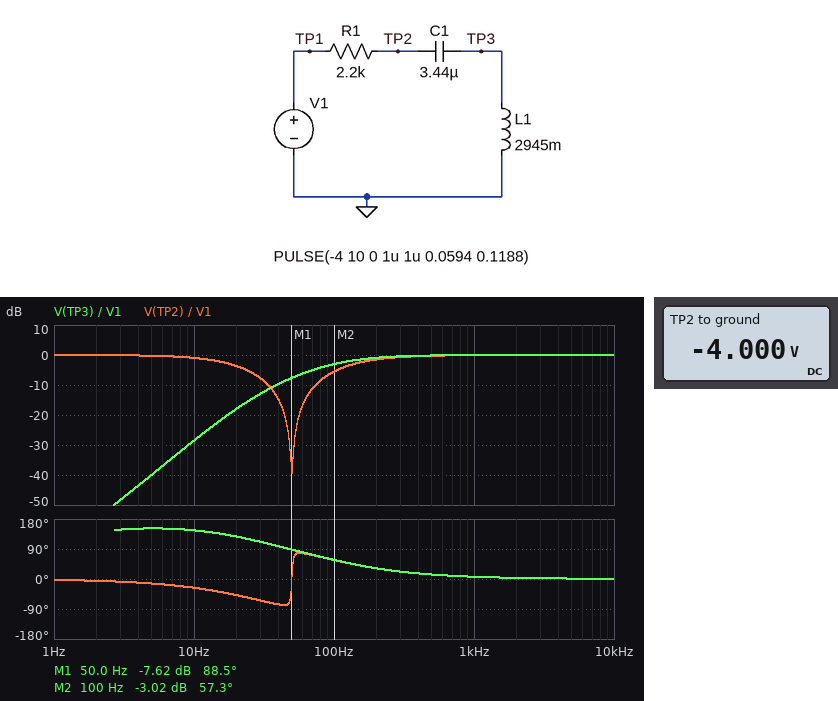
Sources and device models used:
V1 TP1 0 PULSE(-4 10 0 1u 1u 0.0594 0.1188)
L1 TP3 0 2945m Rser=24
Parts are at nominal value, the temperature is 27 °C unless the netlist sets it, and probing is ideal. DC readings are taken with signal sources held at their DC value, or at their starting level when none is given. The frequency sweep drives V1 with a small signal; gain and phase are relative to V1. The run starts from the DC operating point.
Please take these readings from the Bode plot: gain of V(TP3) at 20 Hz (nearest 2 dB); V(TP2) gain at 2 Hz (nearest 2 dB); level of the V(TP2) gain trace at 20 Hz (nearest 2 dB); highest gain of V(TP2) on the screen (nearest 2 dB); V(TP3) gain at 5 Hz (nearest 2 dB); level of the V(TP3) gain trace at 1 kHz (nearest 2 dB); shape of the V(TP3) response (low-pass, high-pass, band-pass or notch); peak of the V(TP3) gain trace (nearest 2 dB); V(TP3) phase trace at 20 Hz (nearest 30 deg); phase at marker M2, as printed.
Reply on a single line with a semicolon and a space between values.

-18 dB; 0 dB; -4 dB; 0 dB; -40 dB; 0 dB; high-pass; 0 dB; 120 deg; 57.3 deg
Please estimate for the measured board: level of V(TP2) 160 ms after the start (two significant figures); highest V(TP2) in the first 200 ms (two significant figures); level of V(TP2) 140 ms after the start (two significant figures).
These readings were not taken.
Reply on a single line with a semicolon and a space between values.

10 V; 10 V; 9.3 V
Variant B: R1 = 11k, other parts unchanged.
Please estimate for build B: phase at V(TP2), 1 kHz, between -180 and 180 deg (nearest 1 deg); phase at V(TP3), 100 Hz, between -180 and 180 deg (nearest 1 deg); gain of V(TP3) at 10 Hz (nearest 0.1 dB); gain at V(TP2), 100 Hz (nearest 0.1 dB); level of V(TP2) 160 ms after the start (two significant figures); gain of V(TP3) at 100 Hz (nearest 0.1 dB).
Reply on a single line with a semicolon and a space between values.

31 deg; 82 deg; -36.1 dB; -18.1 dB; 6.0 V; -15.6 dB
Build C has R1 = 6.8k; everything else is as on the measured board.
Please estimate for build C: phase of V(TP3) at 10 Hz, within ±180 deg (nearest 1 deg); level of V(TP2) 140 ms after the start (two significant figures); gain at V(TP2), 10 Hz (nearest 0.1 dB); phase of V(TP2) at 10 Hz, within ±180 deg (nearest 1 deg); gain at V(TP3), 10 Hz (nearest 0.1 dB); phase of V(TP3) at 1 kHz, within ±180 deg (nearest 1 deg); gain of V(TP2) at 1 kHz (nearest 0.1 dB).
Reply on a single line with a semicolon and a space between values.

116 deg; 4.6 V; -5.3 dB; -57 deg; -32.8 dB; 20 deg; -0.6 dB
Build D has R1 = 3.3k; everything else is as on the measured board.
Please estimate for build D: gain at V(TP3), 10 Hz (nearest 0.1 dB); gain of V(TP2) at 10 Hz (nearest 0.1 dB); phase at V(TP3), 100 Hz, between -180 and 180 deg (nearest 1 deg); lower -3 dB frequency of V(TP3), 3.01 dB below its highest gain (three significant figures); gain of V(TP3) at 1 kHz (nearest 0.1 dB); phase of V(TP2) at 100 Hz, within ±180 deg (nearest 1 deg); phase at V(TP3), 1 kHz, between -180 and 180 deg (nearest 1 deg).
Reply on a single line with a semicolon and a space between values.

-29.5 dB; -1.9 dB; 67 deg; 166 Hz; -0.1 dB; 66 deg; 10 deg
